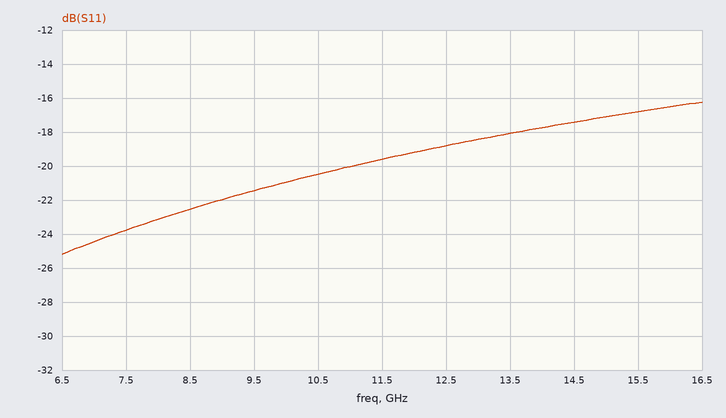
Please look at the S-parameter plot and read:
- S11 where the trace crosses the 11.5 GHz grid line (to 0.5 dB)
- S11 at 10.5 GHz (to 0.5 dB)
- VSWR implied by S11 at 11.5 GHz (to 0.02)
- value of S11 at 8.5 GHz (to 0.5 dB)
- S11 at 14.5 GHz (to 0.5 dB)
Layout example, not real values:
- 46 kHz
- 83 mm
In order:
- -19.5 dB
- -20.5 dB
- 1.24
- -22.5 dB
- -17.5 dB
